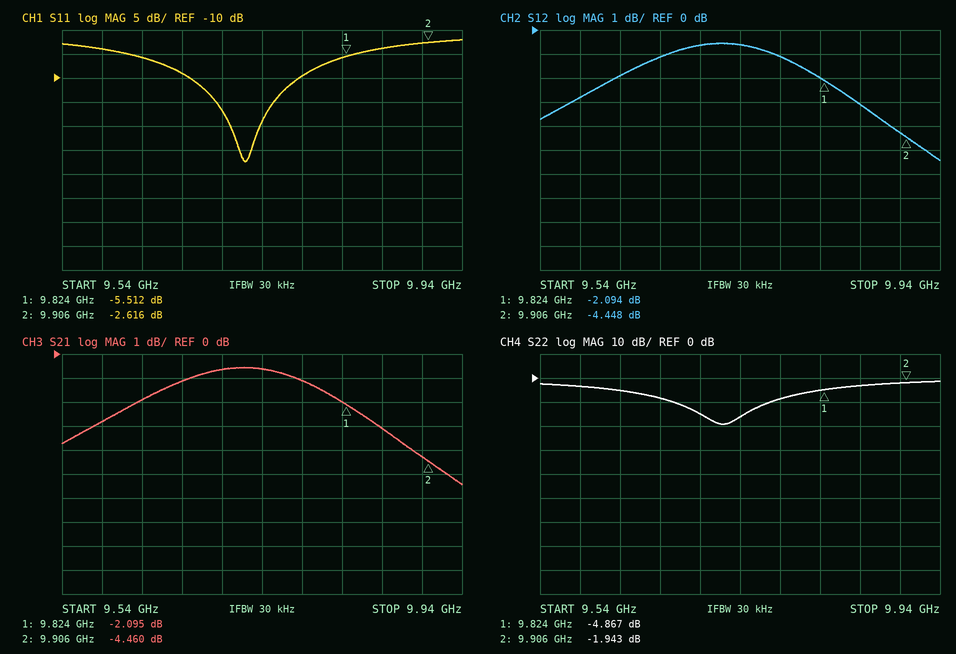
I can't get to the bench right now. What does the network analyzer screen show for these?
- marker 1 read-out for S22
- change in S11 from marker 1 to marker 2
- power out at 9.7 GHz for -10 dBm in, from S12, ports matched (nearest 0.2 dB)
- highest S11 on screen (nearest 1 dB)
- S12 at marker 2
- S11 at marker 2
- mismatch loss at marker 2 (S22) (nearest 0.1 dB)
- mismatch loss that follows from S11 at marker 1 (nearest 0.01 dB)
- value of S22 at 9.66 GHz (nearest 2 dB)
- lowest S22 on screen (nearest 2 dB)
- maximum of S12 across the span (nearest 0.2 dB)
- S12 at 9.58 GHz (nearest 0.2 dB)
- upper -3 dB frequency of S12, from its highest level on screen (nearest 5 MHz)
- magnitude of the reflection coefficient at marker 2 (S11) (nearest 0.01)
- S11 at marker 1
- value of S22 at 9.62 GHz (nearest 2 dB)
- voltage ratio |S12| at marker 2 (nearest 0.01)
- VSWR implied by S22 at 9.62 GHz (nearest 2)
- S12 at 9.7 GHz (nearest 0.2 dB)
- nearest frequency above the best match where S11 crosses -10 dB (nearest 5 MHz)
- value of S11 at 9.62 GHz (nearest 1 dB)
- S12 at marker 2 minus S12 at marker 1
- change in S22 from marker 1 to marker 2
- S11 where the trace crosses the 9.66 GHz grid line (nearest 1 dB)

-4.867 dB
2.896 dB
-10.6 dBm
-2 dB
-4.448 dB
-2.616 dB
4.4 dB
1.43 dB
-8 dB
-20 dB
-0.6 dB
-2.8 dB
9.875 GHz
0.74
-5.512 dB
-6 dB
0.60
4
-0.6 dB
9.775 GHz
-6 dB
-2.354 dB
2.924 dB
-9 dB
